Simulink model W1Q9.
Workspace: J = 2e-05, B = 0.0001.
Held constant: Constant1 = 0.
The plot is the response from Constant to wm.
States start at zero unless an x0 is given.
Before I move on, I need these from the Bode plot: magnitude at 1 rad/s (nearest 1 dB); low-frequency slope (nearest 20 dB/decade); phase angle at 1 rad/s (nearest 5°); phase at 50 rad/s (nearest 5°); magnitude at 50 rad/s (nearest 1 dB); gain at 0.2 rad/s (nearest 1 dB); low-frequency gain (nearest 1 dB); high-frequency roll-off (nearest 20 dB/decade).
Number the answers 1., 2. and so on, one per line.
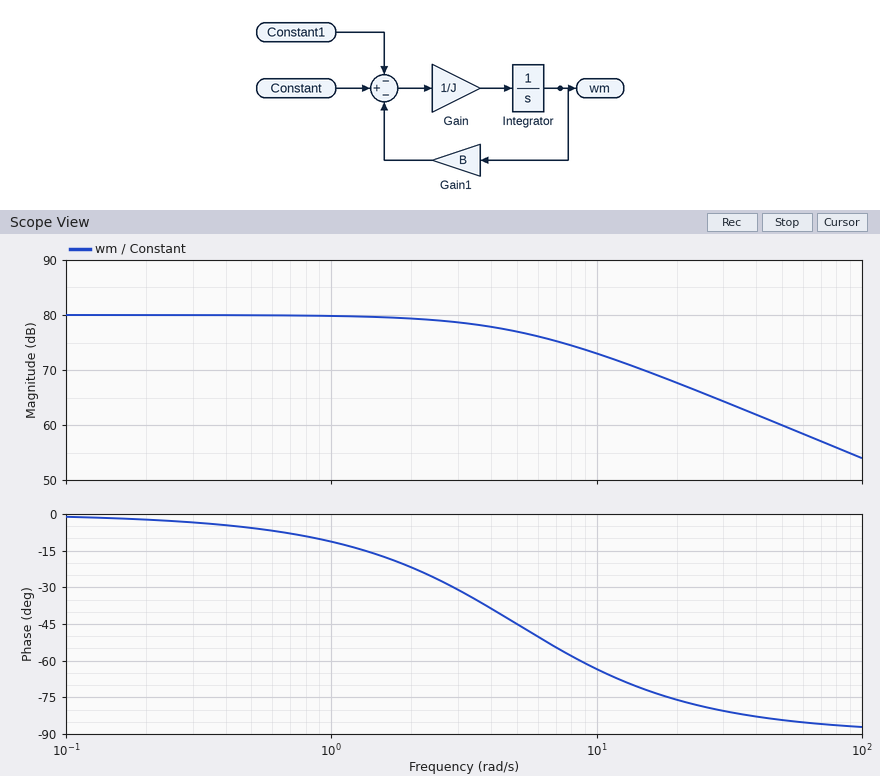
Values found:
1. 80 dB
2. 0 dB/decade
3. -10°
4. -85°
5. 60 dB
6. 80 dB
7. 80 dB
8. -20 dB/decade
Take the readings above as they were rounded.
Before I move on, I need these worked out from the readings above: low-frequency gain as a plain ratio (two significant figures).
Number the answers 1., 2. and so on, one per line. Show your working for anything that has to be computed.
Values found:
1. 10^(80 / 20) = 10000
